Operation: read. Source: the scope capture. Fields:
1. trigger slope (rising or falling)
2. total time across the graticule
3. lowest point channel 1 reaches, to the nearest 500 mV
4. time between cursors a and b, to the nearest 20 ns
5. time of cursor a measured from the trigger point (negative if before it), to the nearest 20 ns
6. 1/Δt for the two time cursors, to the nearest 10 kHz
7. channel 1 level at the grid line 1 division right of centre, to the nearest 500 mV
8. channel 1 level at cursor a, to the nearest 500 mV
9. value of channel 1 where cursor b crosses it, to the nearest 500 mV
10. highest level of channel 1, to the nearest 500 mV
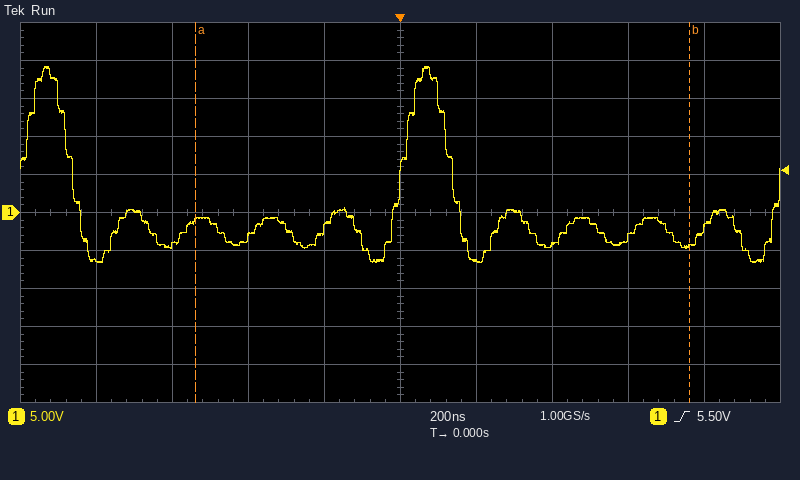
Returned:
rising
2 µs
-6.5 V
1.30 µs
-540 ns
770 kHz
-6.5 V
-1.0 V
-4.5 V
19.0 V
